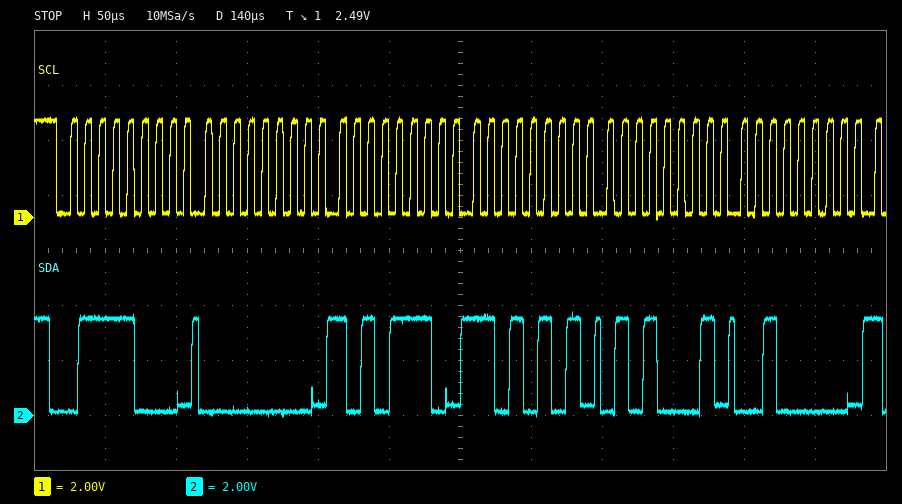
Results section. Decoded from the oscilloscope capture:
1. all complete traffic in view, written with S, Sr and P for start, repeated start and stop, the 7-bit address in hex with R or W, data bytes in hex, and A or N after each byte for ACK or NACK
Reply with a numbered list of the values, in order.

1. S 3CW A 00 A AE A D5 A 51 A 20 A
